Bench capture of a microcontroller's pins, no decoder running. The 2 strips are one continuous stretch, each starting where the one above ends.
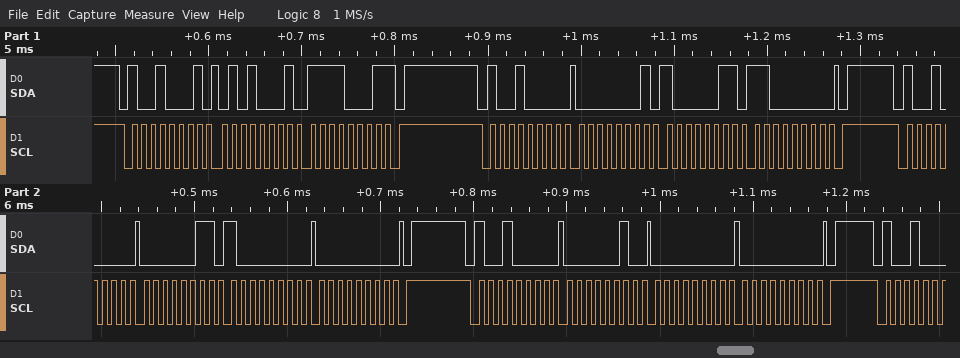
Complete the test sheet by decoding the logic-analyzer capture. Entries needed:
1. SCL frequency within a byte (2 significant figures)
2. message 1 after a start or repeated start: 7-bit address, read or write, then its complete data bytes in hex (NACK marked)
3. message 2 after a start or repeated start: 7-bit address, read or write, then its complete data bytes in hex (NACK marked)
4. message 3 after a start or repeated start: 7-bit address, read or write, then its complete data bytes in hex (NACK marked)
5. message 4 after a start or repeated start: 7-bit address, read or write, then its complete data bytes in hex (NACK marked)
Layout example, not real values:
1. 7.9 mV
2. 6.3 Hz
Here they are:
1. 100 kHz
2. 0x48 read: 51 F1 NACK
3. 0x48 write: 01 83 C0
4. 0x48 write: 03 80 00
5. 0x48 write: 02 00 00
